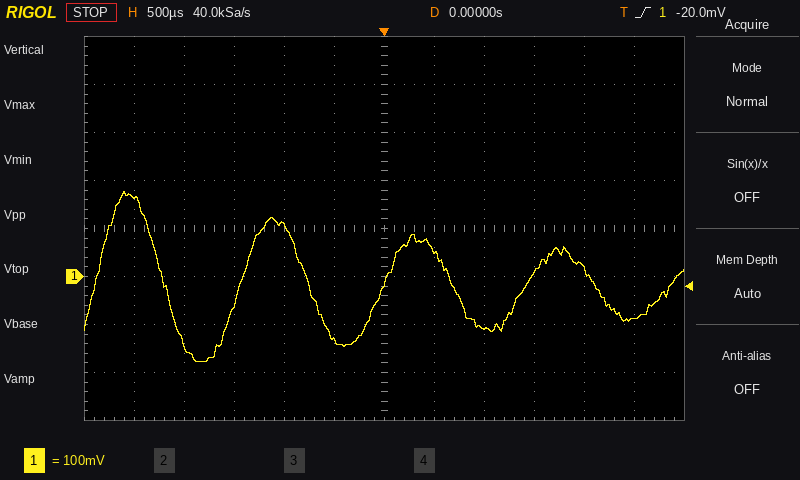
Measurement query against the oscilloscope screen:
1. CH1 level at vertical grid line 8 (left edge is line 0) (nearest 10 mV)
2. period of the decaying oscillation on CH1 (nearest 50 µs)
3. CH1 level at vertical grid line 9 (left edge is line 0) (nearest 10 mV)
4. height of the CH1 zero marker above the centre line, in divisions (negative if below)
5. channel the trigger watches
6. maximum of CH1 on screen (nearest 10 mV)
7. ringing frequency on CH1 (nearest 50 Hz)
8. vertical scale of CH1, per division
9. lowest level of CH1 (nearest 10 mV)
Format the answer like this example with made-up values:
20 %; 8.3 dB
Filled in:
-110 mV; 1.45 ms; 10 mV; -1.0 div; CH1; 180 mV; 700 Hz; 100 mV; -180 mV
